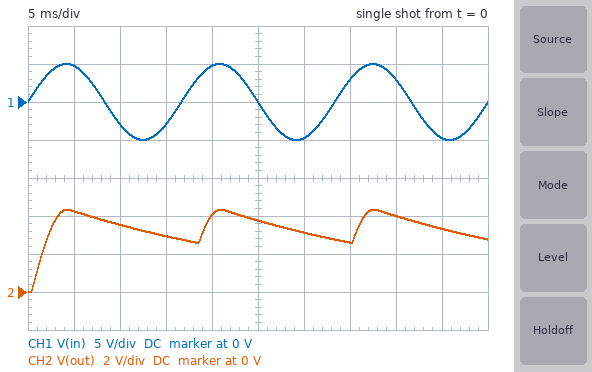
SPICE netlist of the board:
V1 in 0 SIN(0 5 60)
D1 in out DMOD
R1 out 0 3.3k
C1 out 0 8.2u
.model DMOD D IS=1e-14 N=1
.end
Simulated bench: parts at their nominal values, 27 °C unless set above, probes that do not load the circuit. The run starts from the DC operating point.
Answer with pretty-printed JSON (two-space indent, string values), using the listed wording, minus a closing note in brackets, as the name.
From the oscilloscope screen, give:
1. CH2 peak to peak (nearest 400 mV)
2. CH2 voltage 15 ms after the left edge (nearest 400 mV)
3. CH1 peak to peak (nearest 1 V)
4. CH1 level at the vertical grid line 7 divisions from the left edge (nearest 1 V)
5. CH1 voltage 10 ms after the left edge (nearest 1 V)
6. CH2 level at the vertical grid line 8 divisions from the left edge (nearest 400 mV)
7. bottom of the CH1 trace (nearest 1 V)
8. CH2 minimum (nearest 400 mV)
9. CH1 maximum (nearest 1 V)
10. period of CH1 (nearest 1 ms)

{
  "CH2 peak to peak": "4.4 V",
  "CH2 voltage 15 ms after the left edge": "2.8 V",
  "CH1 peak to peak": "10 V",
  "CH1 level at the vertical grid line 7 divisions from the left edge": "3 V",
  "CH1 voltage 10 ms after the left edge": "-3 V",
  "CH2 level at the vertical grid line 8 divisions from the left edge": "4.0 V",
  "bottom of the CH1 trace": "-5 V",
  "CH2 minimum": "0 V",
  "CH1 maximum": "5 V",
  "period of CH1": "17 ms"
}
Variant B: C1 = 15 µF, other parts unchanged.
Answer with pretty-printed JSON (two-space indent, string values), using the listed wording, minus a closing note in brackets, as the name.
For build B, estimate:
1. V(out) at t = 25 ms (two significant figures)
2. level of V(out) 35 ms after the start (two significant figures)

{
  "V(out) at t = 25 ms": "4.0 V",
  "level of V(out) 35 ms after the start": "3.3 V"
}
